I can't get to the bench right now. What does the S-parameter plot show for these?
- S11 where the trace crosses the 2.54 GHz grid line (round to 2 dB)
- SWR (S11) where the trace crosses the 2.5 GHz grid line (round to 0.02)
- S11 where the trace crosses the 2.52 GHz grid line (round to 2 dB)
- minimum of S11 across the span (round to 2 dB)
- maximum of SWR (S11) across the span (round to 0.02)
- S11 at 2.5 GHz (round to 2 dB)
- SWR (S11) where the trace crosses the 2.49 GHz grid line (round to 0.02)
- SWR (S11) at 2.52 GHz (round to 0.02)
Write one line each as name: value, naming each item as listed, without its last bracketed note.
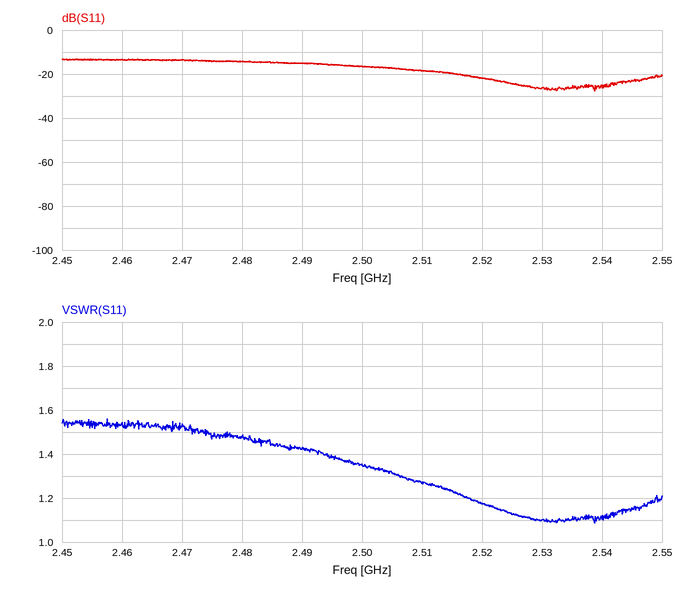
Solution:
S11 where the trace crosses the 2.54 GHz grid line: -26 dB
SWR (S11) where the trace crosses the 2.5 GHz grid line: 1.36
S11 where the trace crosses the 2.52 GHz grid line: -22 dB
minimum of S11 across the span: -28 dB
maximum of SWR (S11) across the span: 1.56
S11 at 2.5 GHz: -16 dB
SWR (S11) where the trace crosses the 2.49 GHz grid line: 1.42
SWR (S11) at 2.52 GHz: 1.18
